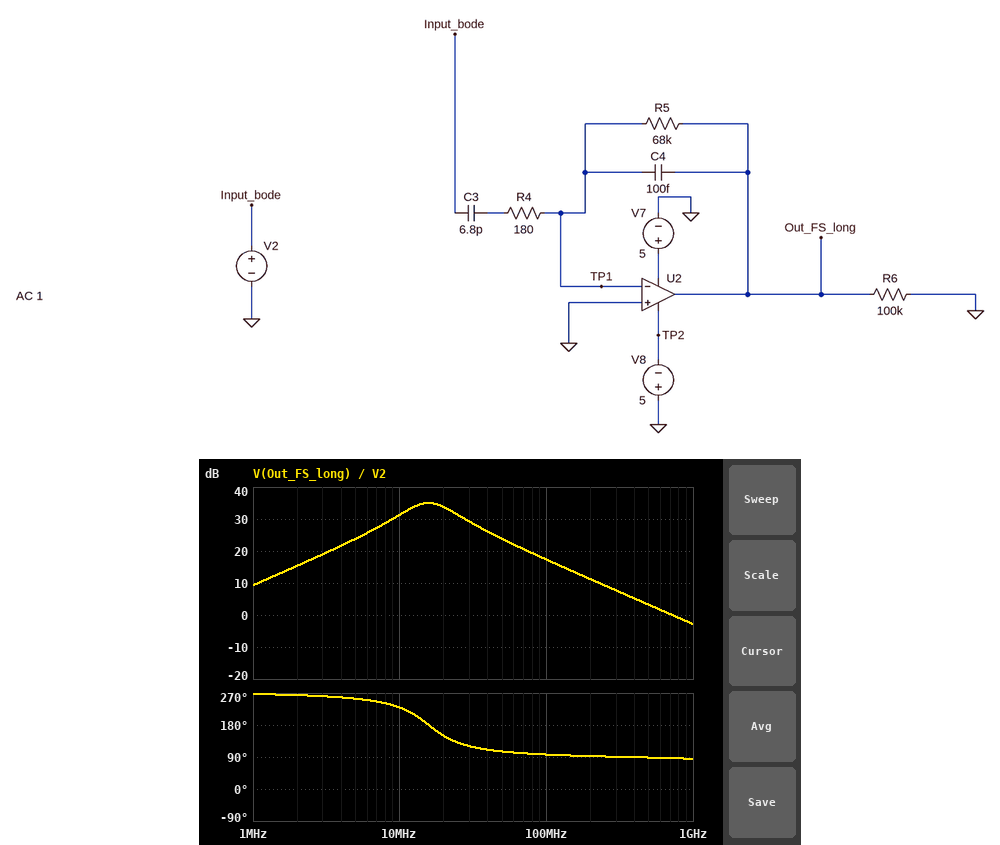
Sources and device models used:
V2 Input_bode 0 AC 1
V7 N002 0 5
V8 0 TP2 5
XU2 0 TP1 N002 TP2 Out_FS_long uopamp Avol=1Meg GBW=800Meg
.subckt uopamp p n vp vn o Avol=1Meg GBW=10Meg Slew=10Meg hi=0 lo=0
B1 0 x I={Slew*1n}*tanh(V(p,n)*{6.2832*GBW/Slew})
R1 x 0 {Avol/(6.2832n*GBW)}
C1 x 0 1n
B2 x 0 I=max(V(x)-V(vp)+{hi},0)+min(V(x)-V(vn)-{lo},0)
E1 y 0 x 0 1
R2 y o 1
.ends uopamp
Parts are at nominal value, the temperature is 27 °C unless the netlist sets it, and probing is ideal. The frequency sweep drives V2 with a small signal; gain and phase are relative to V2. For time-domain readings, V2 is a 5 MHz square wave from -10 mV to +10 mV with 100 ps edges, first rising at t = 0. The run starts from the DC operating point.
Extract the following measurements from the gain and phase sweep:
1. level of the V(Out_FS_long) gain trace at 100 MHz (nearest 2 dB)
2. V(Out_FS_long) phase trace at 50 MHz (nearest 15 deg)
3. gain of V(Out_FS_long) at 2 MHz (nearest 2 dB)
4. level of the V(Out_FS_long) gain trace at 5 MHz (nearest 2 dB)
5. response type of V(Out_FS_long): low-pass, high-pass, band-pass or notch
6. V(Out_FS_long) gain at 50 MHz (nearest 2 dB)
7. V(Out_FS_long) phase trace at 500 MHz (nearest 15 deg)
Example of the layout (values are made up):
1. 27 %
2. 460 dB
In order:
1. 18 dB
2. 105 deg
3. 16 dB
4. 24 dB
5. band-pass
6. 24 dB
7. 90 deg
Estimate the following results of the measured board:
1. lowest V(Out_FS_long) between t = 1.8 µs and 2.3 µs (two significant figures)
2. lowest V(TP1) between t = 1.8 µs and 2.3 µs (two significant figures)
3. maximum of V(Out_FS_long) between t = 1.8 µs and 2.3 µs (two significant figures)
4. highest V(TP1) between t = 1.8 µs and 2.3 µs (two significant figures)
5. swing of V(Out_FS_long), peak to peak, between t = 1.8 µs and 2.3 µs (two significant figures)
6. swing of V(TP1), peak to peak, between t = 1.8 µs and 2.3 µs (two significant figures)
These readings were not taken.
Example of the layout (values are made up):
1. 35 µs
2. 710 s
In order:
1. -320 mV
2. -17 mV
3. 320 mV
4. 17 mV
5. 650 mV
6. 34 mV
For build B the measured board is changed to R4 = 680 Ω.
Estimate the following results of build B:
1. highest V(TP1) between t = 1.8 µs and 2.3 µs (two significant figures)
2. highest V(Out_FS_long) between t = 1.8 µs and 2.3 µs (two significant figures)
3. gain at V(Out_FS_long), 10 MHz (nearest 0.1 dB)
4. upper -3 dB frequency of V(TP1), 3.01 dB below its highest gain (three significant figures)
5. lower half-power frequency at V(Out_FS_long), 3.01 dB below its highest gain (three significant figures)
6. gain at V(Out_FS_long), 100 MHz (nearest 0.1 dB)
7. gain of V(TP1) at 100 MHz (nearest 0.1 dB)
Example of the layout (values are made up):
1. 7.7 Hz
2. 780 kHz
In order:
1. 18 mV
2. 300 mV
3. 30.3 dB
4. 2.40 GHz
5. 8.66 MHz
6. 15.5 dB
7. -2.6 dB
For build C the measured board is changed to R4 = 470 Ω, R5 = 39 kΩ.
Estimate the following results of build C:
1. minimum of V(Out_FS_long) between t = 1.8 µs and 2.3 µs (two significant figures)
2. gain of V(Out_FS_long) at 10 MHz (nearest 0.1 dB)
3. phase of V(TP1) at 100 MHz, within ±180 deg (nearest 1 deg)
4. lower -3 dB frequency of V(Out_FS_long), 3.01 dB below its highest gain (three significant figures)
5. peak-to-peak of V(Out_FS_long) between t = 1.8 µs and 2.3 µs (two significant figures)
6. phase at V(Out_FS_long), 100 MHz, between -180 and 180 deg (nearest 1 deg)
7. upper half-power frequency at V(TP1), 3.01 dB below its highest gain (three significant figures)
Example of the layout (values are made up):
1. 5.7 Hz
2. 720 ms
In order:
1. -240 mV
2. 25.7 dB
3. 9 deg
4. 12.7 MHz
5. 480 mV
6. 99 deg
7. 2.22 GHz
